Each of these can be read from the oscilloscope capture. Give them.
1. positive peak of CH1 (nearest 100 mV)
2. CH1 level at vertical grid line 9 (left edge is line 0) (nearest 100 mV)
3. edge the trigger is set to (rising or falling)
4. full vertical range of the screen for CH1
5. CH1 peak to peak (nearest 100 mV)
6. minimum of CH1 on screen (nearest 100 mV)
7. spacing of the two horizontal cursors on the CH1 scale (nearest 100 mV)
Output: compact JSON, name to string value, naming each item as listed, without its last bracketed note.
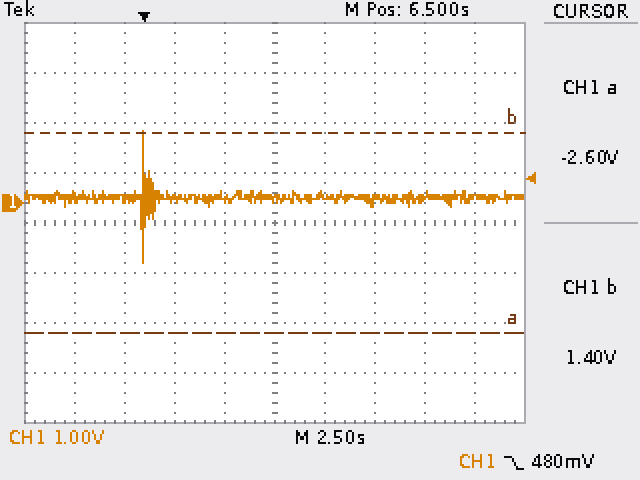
{"positive peak of CH1": "1.4 V", "CH1 level at vertical grid line 9 (left edge is line 0)": "100 mV", "edge the trigger is set to": "falling", "full vertical range of the screen for CH1": "8 V", "CH1 peak to peak": "2.6 V", "minimum of CH1 on screen": "-1.2 V", "spacing of the two horizontal cursors on the CH1 scale": "4.0 V"}
